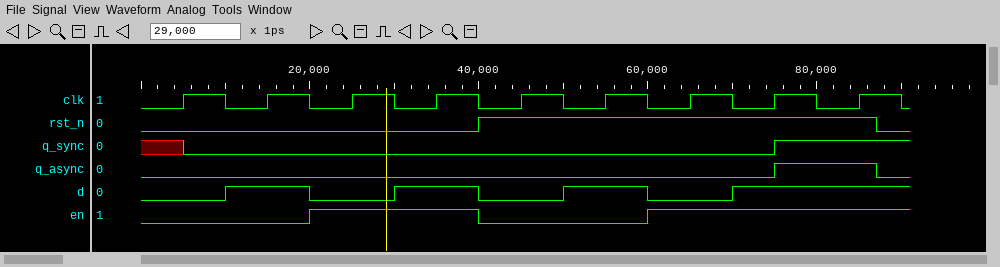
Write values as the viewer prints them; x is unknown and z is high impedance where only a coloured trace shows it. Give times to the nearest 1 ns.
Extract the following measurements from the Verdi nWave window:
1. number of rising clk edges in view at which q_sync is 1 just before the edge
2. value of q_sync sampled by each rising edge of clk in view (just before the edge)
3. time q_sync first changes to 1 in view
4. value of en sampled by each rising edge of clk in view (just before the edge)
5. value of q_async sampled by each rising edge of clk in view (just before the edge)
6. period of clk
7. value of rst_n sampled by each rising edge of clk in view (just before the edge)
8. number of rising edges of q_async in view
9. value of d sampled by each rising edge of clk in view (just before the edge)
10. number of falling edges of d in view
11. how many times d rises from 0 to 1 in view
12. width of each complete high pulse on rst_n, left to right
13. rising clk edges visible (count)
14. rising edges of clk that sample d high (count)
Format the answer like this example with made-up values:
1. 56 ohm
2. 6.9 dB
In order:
1. 1
2. x 0 0 0 0 0 0 0 1
3. 75 ns
4. 0 0 1 1 0 0 1 1 1
5. 0 0 0 0 0 0 0 0 1
6. 10 ns
7. 0 0 0 0 1 1 1 1 1
8. 1
9. 0 1 0 1 0 1 0 1 1
10. 3
11. 4
12. 47 ns
13. 9
14. 5
